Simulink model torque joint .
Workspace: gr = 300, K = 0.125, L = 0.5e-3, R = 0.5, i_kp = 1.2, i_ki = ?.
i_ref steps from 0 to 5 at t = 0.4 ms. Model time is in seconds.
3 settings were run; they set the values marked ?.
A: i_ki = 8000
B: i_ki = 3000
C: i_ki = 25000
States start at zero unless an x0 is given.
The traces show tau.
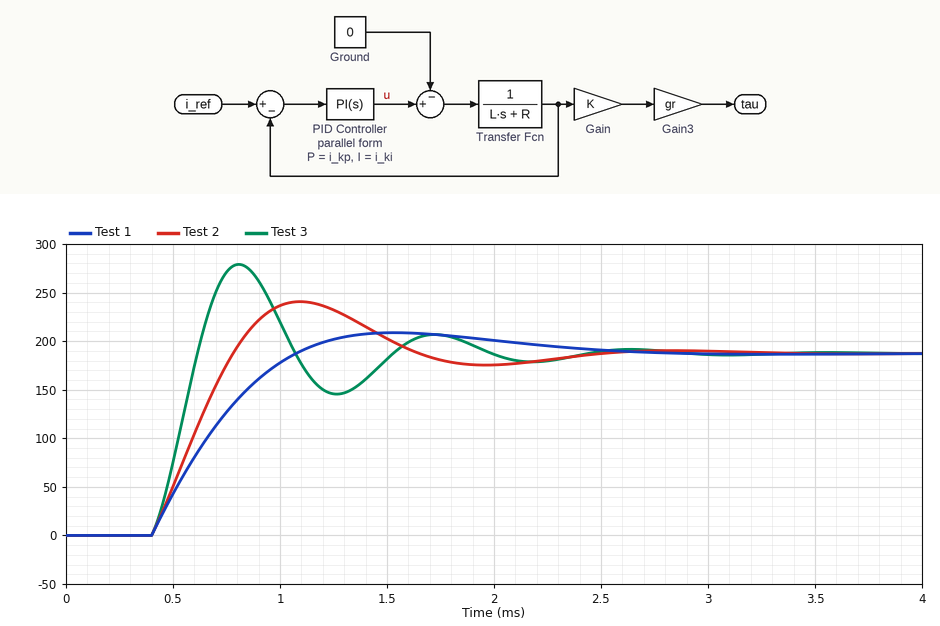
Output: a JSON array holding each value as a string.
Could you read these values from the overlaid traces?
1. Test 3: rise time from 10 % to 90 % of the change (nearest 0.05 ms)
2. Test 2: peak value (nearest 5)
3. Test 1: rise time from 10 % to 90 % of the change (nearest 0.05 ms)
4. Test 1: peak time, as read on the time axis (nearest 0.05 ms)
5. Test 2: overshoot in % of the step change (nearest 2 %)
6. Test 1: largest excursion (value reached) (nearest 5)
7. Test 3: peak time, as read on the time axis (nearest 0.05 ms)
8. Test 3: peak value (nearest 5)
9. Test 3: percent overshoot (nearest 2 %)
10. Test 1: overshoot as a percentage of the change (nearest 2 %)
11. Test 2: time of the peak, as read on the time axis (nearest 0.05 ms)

["0.15 ms", "240", "0.50 ms", "1.55 ms", "28 %", "210", "0.80 ms", "280", "48 %", "12 %", "1.10 ms"]
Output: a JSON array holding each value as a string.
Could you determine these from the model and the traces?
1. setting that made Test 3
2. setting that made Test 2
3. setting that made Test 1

["C", "A", "B"]
